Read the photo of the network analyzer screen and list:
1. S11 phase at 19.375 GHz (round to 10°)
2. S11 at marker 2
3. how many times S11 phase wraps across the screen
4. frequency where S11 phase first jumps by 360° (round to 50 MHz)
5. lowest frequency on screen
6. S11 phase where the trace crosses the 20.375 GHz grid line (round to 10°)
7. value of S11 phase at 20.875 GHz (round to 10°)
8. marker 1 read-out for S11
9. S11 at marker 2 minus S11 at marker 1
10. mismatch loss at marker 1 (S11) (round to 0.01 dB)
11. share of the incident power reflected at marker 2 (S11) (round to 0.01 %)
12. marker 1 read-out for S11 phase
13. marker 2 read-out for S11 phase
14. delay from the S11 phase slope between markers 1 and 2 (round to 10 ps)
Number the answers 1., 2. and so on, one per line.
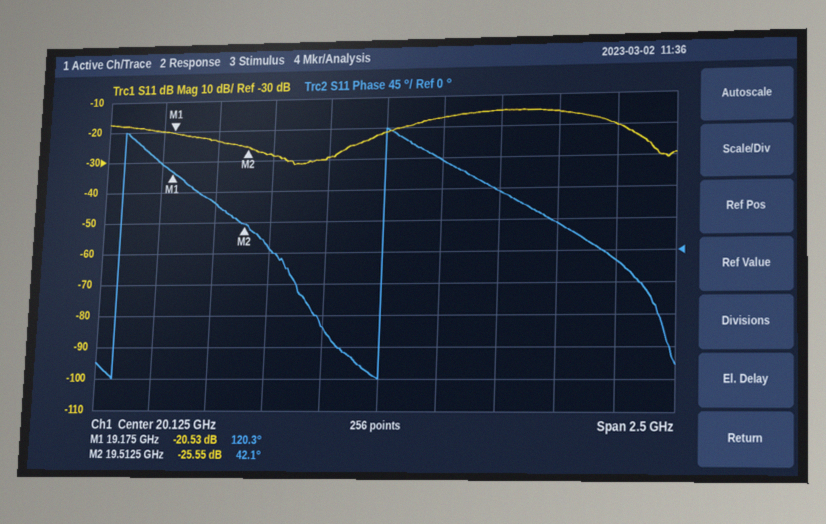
1. 70°
2. -25.55 dB
3. 2
4. 18.95 GHz
5. 18.875 GHz
6. 130°
7. 40°
8. -20.53 dB
9. -5.02 dB
10. 0.04 dB
11. 0.28 %
12. 120.3°
13. 42.1°
14. 640 ps
